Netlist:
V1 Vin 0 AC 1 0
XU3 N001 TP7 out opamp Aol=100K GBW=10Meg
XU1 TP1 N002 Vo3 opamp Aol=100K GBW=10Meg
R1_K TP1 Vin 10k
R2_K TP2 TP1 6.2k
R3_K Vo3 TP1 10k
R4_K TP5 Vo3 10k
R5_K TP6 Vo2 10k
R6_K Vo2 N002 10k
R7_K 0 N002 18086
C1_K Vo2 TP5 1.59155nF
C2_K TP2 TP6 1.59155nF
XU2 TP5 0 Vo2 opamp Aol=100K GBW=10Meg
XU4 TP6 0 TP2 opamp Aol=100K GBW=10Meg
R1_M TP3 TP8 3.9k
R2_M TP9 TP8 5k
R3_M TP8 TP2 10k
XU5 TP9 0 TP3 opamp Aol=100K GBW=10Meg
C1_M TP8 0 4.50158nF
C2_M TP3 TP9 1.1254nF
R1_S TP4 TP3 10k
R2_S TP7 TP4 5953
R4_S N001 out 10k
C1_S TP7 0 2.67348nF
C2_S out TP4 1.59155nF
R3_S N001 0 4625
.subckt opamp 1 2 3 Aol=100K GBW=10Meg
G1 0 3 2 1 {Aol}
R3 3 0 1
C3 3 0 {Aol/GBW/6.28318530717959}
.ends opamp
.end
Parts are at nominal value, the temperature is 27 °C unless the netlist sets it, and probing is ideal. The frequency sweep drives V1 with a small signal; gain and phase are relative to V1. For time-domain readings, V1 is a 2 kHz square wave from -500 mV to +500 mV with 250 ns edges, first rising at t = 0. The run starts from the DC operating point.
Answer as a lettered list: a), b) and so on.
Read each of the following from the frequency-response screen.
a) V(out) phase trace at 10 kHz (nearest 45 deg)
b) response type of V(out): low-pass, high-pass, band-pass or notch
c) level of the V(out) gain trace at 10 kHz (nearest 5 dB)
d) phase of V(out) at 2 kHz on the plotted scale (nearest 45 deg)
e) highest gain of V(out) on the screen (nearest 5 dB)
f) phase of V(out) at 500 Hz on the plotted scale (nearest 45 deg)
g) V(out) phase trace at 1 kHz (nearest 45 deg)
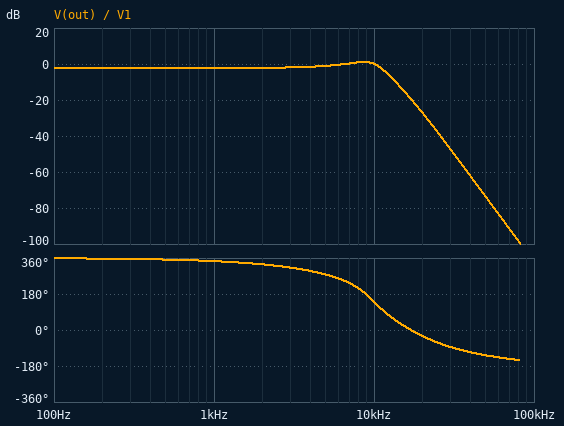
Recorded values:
a) 135 deg
b) low-pass
c) 0 dB
d) 315 deg
e) 0 dB
f) 360 deg
g) 360 deg
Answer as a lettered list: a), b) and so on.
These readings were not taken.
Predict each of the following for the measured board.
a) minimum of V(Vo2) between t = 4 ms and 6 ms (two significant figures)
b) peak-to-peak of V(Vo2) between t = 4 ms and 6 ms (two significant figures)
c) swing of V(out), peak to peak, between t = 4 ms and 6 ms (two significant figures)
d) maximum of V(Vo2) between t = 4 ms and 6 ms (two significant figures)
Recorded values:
a) -310 mV
b) 620 mV
c) 1.2 V
d) 310 mV
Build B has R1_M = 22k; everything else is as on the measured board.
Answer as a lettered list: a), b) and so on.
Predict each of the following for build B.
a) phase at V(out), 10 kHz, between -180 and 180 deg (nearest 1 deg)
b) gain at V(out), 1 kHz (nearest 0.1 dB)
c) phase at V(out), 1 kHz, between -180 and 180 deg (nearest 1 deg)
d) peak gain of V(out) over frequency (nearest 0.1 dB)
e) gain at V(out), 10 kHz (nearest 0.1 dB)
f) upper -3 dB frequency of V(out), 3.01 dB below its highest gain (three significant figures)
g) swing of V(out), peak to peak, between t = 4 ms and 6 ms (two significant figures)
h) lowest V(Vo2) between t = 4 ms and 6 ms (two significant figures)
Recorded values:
a) 79 deg
b) 12.6 dB
c) -27 deg
d) 12.7 dB
e) 5.6 dB
f) 6.78 kHz
g) 4.5 V
h) -310 mV
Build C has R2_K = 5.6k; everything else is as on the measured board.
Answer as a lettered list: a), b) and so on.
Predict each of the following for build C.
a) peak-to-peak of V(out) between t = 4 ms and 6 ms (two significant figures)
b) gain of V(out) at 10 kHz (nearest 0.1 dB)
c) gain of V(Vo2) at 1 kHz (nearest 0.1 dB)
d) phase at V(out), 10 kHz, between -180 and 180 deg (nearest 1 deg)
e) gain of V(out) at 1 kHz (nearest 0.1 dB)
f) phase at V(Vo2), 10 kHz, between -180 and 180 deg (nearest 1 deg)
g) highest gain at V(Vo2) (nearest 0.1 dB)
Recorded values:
a) 1.1 V
b) -0.4 dB
c) -25.1 dB
d) 145 deg
e) -3.2 dB
f) 18 deg
g) -7.7 dB
